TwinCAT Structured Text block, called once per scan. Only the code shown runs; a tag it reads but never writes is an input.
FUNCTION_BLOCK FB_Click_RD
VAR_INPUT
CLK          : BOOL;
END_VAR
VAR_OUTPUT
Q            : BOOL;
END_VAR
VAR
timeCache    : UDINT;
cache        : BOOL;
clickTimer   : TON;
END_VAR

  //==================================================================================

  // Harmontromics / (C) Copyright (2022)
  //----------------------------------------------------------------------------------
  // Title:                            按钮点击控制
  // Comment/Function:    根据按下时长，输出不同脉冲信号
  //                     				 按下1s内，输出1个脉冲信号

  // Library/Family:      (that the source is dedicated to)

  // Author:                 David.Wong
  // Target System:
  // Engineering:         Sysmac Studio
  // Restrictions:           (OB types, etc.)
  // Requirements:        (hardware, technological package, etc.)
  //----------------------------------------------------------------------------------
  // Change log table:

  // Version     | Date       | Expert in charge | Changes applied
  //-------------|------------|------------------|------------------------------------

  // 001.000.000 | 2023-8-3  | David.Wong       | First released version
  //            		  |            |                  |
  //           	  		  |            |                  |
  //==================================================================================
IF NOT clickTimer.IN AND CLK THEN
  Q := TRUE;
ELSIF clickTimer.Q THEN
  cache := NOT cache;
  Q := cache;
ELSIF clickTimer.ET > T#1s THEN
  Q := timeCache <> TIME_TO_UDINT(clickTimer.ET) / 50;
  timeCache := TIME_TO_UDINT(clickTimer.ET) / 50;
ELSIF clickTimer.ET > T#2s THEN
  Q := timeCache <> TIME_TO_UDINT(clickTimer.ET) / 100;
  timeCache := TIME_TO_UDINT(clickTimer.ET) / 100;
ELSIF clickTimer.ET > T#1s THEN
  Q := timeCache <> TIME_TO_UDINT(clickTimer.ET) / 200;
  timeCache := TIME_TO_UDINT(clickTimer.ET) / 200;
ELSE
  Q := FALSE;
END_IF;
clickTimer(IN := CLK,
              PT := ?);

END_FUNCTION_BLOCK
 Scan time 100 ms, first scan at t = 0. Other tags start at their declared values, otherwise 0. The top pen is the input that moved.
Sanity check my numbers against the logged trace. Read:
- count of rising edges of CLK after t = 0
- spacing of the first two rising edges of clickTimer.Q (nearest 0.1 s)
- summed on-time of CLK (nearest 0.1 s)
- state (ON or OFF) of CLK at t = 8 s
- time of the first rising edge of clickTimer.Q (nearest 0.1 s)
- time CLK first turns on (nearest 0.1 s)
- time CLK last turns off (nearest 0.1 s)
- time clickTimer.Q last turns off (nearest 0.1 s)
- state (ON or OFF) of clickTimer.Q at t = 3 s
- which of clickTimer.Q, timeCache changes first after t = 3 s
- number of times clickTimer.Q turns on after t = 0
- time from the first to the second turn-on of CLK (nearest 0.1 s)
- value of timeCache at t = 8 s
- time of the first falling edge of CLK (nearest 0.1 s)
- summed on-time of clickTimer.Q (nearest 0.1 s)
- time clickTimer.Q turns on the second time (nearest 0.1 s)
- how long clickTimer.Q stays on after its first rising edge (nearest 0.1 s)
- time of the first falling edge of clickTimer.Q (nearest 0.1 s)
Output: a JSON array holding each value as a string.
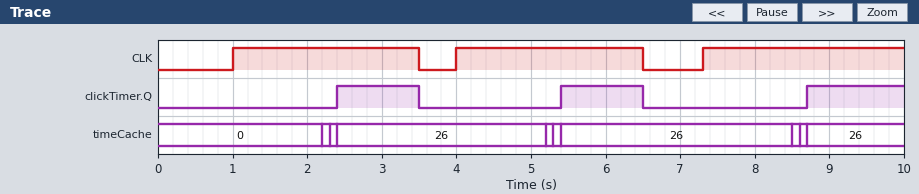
["3", "3.0 s", "7.7 s", "ON", "2.4 s", "1.0 s", "6.5 s", "6.5 s", "ON", "clickTimer.Q", "3", "3.0 s", "26", "3.5 s", "3.5 s", "5.4 s", "1.1 s", "3.5 s"]
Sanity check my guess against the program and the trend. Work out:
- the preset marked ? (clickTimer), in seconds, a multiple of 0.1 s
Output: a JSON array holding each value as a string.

["1.4 s"]
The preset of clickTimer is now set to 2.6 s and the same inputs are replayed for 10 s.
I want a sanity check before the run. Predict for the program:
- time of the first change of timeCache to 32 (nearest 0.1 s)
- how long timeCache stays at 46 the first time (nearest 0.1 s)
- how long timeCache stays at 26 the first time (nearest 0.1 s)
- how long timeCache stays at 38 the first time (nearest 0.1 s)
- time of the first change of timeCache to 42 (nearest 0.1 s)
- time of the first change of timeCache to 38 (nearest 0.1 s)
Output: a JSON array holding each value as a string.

["2.7 s", "0.1 s", "0.1 s", "0.1 s", "3.2 s", "3.0 s"]
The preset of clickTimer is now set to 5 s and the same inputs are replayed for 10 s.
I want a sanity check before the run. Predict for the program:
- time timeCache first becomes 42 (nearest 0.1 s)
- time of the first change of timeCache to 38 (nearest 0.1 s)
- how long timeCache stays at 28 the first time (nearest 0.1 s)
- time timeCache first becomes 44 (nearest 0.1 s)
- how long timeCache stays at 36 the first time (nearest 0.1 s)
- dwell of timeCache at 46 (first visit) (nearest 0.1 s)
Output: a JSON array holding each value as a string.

["3.2 s", "3.0 s", "0.1 s", "3.3 s", "0.1 s", "0.1 s"]
